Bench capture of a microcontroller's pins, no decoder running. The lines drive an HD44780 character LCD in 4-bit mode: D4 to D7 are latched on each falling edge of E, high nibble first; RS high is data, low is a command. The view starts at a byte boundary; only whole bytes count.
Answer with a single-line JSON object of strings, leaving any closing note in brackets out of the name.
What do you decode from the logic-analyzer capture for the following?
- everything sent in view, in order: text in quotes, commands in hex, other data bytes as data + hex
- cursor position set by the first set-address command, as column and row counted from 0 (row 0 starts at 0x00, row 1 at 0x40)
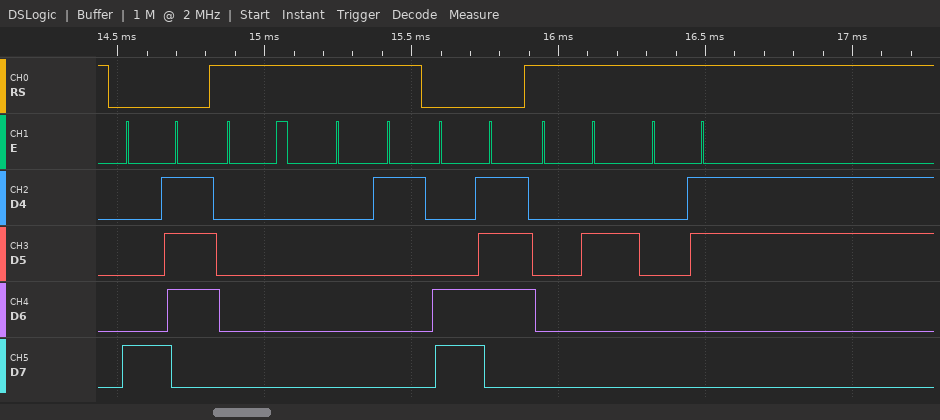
{"everything sent in view, in order: text in quotes, commands in hex, other data bytes as data + hex": "0x87 data 00 01 0xC7 data 02 03", "cursor position set by the first set-address command, as column and row counted from 0": "column 7, row 0"}
